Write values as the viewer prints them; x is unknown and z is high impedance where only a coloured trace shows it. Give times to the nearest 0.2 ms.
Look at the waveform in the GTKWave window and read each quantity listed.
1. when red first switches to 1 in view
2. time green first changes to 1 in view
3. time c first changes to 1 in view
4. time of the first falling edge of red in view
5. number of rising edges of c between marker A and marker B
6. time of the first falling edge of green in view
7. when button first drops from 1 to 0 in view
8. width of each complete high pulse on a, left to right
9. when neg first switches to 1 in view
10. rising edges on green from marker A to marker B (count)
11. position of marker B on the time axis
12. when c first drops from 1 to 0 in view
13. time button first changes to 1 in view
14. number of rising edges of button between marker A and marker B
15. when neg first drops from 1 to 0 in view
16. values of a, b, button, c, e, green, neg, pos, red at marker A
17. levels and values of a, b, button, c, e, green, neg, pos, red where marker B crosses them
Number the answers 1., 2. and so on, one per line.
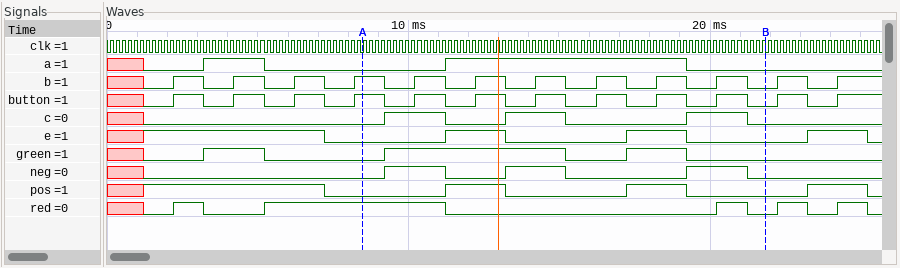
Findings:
1. 2.2 ms
2. 3.2 ms
3. 9.2 ms
4. 3.2 ms
5. 3
6. 5.2 ms
7. 3.2 ms
8. 2 ms, 8 ms
9. 9.2 ms
10. 2
11. 21.8 ms
12. 11.2 ms
13. 2.2 ms
14. 6
15. 11.2 ms
16. a=0, b=1, button=1, c=0, e=0, green=0, neg=0, pos=0, red=1
17. a=0, b=0, button=0, c=0, e=0, green=0, neg=0, pos=0, red=0
